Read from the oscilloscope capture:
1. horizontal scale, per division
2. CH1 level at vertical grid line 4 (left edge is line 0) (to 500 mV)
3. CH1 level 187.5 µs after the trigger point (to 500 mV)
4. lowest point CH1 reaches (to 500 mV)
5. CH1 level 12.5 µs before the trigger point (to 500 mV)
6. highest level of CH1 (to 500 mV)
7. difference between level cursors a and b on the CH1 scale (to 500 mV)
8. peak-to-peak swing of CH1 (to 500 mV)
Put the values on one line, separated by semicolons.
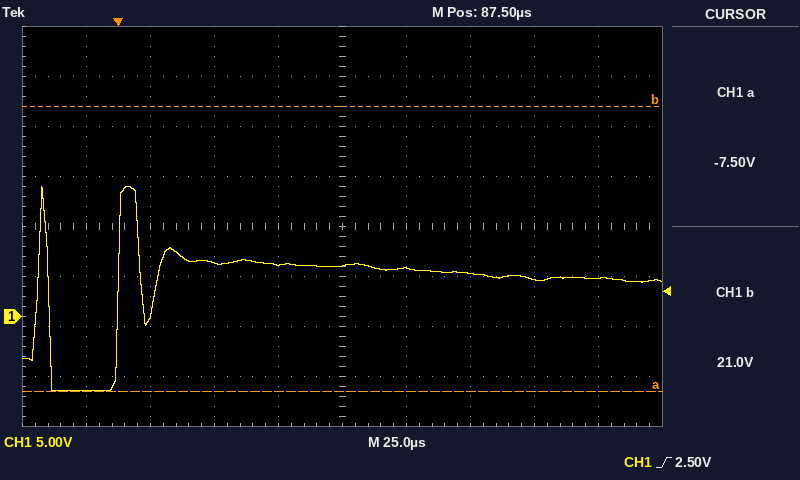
25 µs; 5.0 V; 4.0 V; -7.5 V; -7.5 V; 13.0 V; 28.5 V; 20.5 V
